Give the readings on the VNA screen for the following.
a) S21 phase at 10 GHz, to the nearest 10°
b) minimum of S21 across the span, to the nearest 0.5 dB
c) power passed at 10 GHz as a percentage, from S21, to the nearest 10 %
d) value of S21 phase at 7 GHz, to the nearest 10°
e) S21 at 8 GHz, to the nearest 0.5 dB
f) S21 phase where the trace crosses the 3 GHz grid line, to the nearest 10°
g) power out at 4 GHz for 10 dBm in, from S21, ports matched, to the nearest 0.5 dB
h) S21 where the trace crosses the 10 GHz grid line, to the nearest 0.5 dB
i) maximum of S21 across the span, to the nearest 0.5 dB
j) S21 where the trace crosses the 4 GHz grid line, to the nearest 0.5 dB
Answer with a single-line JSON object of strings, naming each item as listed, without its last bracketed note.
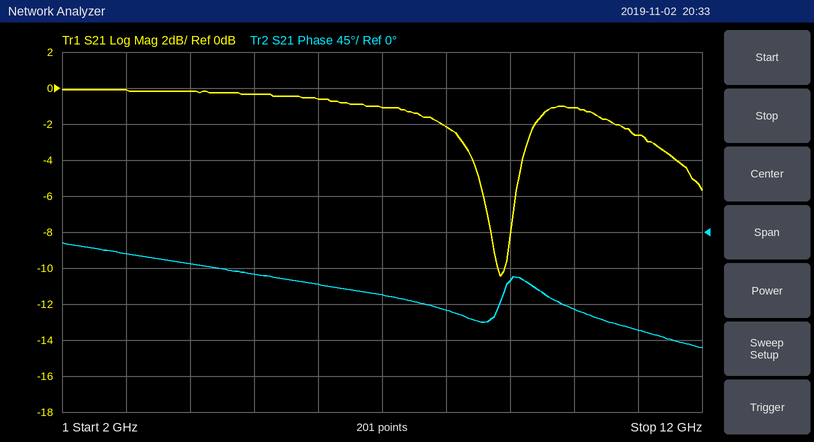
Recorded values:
{"S21 phase at 10 GHz, to the nearest 10°": "-100°", "minimum of S21 across the span, to the nearest 0.5 dB": "-10.5 dB", "power passed at 10 GHz as a percentage, from S21, to the nearest 10 %": "80 %", "value of S21 phase at 7 GHz, to the nearest 10°": "-80°", "S21 at 8 GHz, to the nearest 0.5 dB": "-2.0 dB", "S21 phase where the trace crosses the 3 GHz grid line, to the nearest 10°": "-30°", "power out at 4 GHz for 10 dBm in, from S21, ports matched, to the nearest 0.5 dB": "10.0 dBm", "S21 where the trace crosses the 10 GHz grid line, to the nearest 0.5 dB": "-1.0 dB", "maximum of S21 across the span, to the nearest 0.5 dB": "0.0 dB", "S21 where the trace crosses the 4 GHz grid line, to the nearest 0.5 dB": "0.0 dB"}
